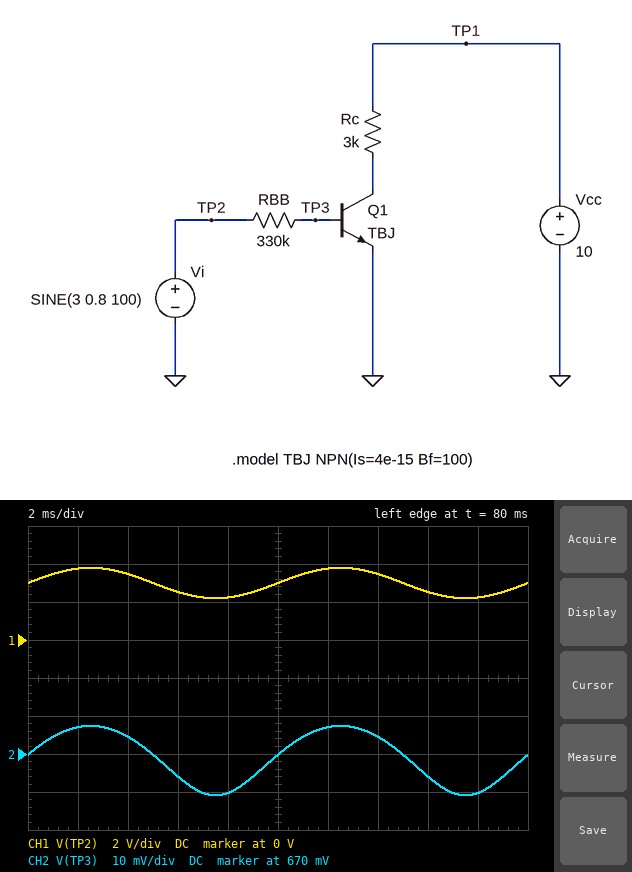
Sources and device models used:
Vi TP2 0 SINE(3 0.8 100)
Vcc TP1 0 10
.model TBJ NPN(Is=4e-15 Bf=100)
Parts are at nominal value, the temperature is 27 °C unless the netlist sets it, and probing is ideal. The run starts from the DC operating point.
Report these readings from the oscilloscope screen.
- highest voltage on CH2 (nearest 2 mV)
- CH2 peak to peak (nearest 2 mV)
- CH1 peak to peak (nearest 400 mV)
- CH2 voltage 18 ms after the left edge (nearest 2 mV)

678 mV
18 mV
1.6 V
660 mV
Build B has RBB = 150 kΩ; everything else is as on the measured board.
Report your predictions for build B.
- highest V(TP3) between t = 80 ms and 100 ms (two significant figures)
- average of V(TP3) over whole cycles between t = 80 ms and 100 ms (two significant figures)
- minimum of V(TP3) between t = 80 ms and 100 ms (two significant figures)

700 mV
690 mV
680 mV
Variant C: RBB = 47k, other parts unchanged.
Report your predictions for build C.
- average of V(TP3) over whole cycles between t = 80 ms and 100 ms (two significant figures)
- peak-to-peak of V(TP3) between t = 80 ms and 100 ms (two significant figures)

710 mV
1.5 mV
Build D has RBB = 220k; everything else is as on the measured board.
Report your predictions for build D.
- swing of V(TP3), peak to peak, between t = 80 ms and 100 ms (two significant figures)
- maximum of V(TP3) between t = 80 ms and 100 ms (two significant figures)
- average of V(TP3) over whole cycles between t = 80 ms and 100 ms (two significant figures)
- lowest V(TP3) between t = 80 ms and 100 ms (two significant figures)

18 mV
690 mV
680 mV
670 mV
